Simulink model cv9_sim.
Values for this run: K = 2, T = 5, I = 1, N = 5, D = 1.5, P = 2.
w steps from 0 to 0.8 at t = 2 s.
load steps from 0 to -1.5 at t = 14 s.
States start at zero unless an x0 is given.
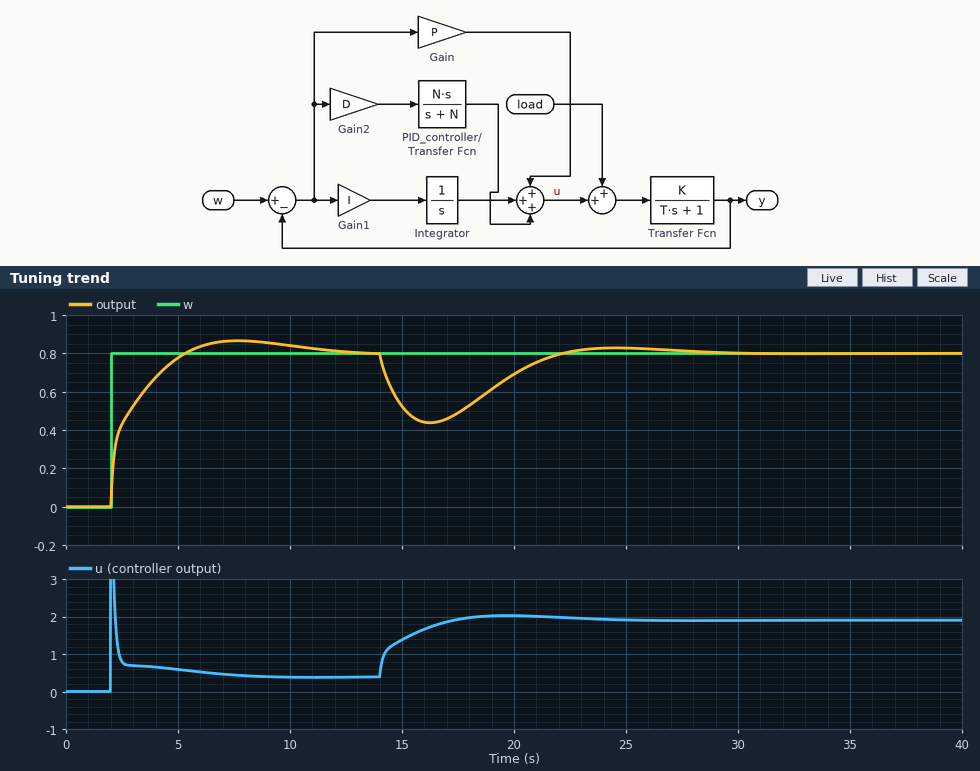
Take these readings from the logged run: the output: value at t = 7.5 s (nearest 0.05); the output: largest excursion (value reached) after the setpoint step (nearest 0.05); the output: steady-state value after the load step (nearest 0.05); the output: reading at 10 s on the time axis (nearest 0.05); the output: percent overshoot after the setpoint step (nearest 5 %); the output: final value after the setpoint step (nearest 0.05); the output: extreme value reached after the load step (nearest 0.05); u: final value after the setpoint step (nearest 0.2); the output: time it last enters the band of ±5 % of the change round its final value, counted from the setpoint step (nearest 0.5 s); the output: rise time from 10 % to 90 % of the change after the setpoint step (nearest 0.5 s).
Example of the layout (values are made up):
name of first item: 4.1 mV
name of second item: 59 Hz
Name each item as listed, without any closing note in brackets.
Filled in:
the output: value at t = 7.5 s: 0.85
the output: largest excursion (value reached) after the setpoint step: 0.85
the output: steady-state value after the load step: 0.80
the output: reading at 10 s on the time axis: 0.85
the output: percent overshoot after the setpoint step: 10 %
the output: final value after the setpoint step: 0.80
the output: extreme value reached after the load step: 0.45
u: final value after the setpoint step: 0.4
the output: time it last enters the band of ±5 % of the change round its final value, counted from the setpoint step: 8.0 s
the output: rise time from 10 % to 90 % of the change after the setpoint step: 2.5 s
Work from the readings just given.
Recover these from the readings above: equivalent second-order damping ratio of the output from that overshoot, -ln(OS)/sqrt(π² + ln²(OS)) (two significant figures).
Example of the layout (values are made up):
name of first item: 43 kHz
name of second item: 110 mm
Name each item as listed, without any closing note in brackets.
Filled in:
equivalent second-order damping ratio of the output from that overshoot, -ln(OS)/sqrt(π² + ln²(OS)): 0.59
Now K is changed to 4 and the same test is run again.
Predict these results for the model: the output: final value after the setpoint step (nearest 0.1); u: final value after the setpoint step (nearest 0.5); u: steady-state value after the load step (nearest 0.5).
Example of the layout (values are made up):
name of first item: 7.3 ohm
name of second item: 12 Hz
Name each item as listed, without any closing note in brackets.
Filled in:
the output: final value after the setpoint step: 0.8
u: final value after the setpoint step: 0.0
u: steady-state value after the load step: 1.5
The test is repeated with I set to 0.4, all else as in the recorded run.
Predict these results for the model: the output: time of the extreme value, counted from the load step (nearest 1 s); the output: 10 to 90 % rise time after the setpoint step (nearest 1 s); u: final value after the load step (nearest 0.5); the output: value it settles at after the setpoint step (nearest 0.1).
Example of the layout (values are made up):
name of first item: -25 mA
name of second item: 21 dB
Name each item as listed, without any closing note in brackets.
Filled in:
the output: time of the extreme value, counted from the load step: 3 s
the output: 10 to 90 % rise time after the setpoint step: 4 s
u: final value after the load step: 2.0
the output: value it settles at after the setpoint step: 0.8
